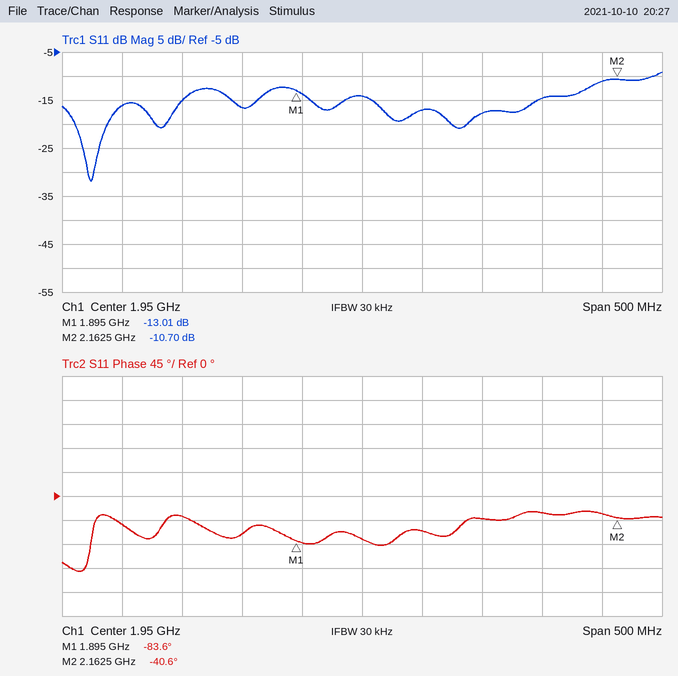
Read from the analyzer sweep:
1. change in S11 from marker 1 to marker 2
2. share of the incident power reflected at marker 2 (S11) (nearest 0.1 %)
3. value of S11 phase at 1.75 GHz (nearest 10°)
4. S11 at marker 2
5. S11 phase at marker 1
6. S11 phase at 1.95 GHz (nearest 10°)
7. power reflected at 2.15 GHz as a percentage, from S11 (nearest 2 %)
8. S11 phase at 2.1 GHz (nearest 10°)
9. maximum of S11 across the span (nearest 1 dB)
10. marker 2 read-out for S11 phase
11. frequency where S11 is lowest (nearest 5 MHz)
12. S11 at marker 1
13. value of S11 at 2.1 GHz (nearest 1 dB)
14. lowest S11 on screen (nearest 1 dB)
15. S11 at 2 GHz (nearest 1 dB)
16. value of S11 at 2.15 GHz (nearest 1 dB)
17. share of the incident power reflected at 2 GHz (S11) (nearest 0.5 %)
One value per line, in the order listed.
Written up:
2.31 dB
8.5 %
-50°
-10.70 dB
-83.6°
-80°
8 %
-30°
-9 dB
-40.6°
1.725 GHz
-13.01 dB
-15 dB
-32 dB
-17 dB
-11 dB
2.0 %
